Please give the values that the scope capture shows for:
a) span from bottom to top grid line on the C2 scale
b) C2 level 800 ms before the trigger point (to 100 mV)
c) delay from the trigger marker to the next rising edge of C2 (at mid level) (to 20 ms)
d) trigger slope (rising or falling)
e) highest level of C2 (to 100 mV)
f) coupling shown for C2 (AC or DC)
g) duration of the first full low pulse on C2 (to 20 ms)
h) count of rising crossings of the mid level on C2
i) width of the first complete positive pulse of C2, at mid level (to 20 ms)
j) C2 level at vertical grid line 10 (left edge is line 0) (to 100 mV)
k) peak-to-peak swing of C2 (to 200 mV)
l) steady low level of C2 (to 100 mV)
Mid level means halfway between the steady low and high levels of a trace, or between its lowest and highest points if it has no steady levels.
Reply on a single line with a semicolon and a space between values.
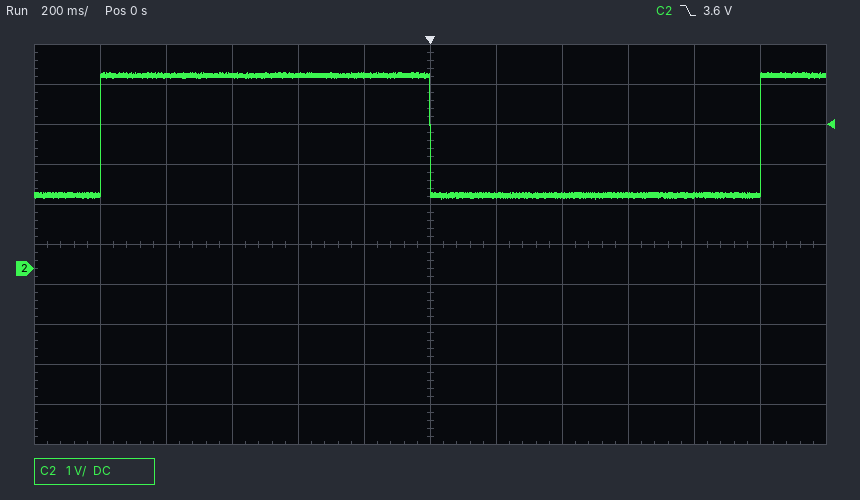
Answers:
10 V; 4.8 V; 1.00 s; falling; 4.9 V; DC; 1.00 s; 2; 1.00 s; 1.8 V; 3.2 V; 1.8 V
